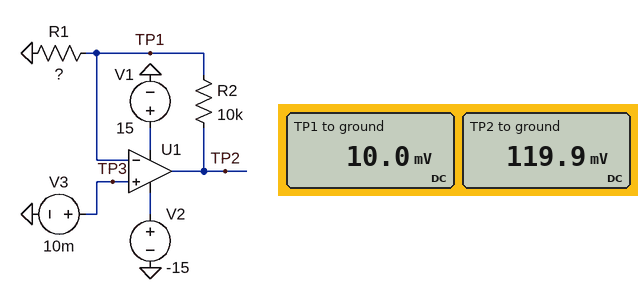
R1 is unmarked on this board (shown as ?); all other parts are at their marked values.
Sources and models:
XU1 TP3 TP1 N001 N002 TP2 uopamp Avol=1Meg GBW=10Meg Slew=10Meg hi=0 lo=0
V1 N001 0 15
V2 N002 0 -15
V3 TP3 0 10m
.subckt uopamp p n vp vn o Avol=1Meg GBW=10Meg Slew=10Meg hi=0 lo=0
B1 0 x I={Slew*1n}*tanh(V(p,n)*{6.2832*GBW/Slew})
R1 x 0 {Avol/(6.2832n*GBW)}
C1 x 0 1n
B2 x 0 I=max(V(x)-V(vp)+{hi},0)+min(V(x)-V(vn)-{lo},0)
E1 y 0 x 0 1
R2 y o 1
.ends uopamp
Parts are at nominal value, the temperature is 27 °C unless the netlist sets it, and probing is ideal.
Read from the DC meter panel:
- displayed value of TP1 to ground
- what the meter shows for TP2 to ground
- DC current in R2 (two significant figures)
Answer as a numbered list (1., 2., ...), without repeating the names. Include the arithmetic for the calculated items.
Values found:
1. 10.0 mV
2. 119.9 mV
3. (119.9 mV - 10 mV) / 10 kΩ = 11 µA
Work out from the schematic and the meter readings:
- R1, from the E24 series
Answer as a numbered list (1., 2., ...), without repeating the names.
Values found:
1. 910 Ω
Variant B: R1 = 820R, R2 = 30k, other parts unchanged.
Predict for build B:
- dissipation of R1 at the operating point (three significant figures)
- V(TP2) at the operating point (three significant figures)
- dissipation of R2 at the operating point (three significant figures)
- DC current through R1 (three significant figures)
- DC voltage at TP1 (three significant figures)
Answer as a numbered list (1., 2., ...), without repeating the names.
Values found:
1. 122 nW
2. 376 mV
3. 4.46 µW
4. 12.2 µA
5. 10.0 mV
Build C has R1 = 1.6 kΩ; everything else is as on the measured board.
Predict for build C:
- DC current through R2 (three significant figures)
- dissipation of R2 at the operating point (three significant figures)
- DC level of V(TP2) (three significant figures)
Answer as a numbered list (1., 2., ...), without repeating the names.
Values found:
1. 6.25 µA
2. 391 nW
3. 72.5 mV
